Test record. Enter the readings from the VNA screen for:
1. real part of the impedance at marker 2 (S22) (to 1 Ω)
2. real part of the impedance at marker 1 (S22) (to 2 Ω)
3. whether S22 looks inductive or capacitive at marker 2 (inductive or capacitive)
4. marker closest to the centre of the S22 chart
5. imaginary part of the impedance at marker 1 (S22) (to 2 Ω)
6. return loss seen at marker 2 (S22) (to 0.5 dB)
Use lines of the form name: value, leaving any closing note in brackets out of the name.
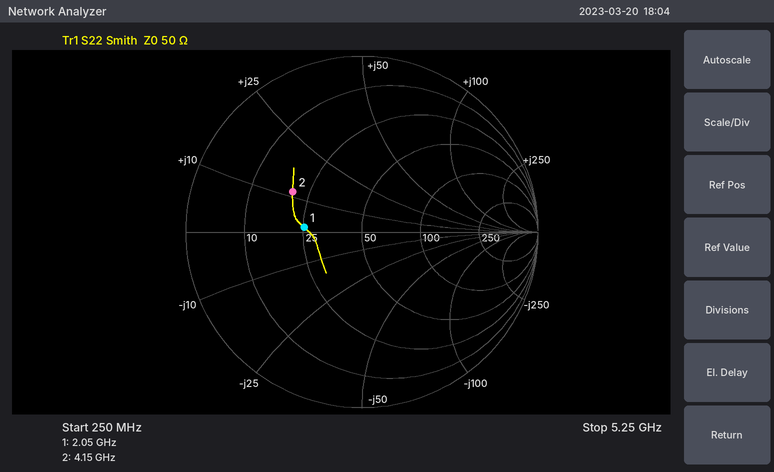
real part of the impedance at marker 2 (S22): 20 Ω
real part of the impedance at marker 1 (S22): 26 Ω
whether S22 looks inductive or capacitive at marker 2: inductive
marker closest to the centre of the S22 chart: marker 1
imaginary part of the impedance at marker 1 (S22): +2 Ω
return loss seen at marker 2 (S22): 7.0 dB
